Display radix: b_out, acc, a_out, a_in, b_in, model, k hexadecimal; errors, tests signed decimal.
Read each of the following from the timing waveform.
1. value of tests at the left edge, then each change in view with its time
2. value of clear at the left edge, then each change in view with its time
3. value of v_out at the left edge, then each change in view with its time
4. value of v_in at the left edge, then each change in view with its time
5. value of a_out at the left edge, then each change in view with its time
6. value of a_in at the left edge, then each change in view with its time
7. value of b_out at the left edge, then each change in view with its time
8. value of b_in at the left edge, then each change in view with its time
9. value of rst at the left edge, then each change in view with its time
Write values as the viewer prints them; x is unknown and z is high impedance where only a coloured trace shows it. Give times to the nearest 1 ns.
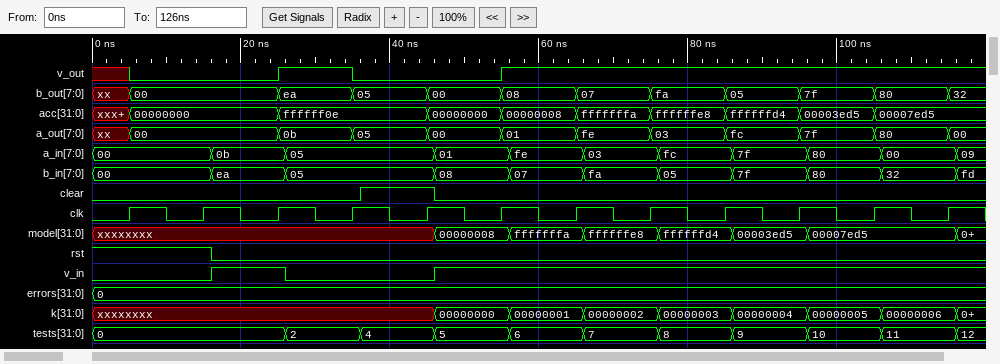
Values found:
0, 2 at 26 ns, 4 at 36 ns, 5 at 46 ns, 6 at 56 ns, 7 at 66 ns, 8 at 76 ns, 9 at 86 ns, 10 at 96 ns, 11 at 106 ns, 12 at 116 ns
0, 1 at 36 ns, 0 at 46 ns
x, 0 at 5 ns, 1 at 25 ns, 0 at 35 ns, 1 at 55 ns
0, 1 at 16 ns, 0 at 26 ns, 1 at 46 ns
xx, 00 at 5 ns, 0b at 25 ns, 05 at 35 ns, 00 at 45 ns, 01 at 55 ns, fe at 65 ns, 03 at 75 ns, fc at 85 ns, 7f at 95 ns, 80 at 105 ns, 00 at 115 ns
00, 0b at 16 ns, 05 at 26 ns, 01 at 46 ns, fe at 56 ns, 03 at 66 ns, fc at 76 ns, 7f at 86 ns, 80 at 96 ns, 00 at 106 ns, 09 at 116 ns
xx, 00 at 5 ns, ea at 25 ns, 05 at 35 ns, 00 at 45 ns, 08 at 55 ns, 07 at 65 ns, fa at 75 ns, 05 at 85 ns, 7f at 95 ns, 80 at 105 ns, 32 at 115 ns
00, ea at 16 ns, 05 at 26 ns, 08 at 46 ns, 07 at 56 ns, fa at 66 ns, 05 at 76 ns, 7f at 86 ns, 80 at 96 ns, 32 at 106 ns, fd at 116 ns
1, 0 at 16 ns
